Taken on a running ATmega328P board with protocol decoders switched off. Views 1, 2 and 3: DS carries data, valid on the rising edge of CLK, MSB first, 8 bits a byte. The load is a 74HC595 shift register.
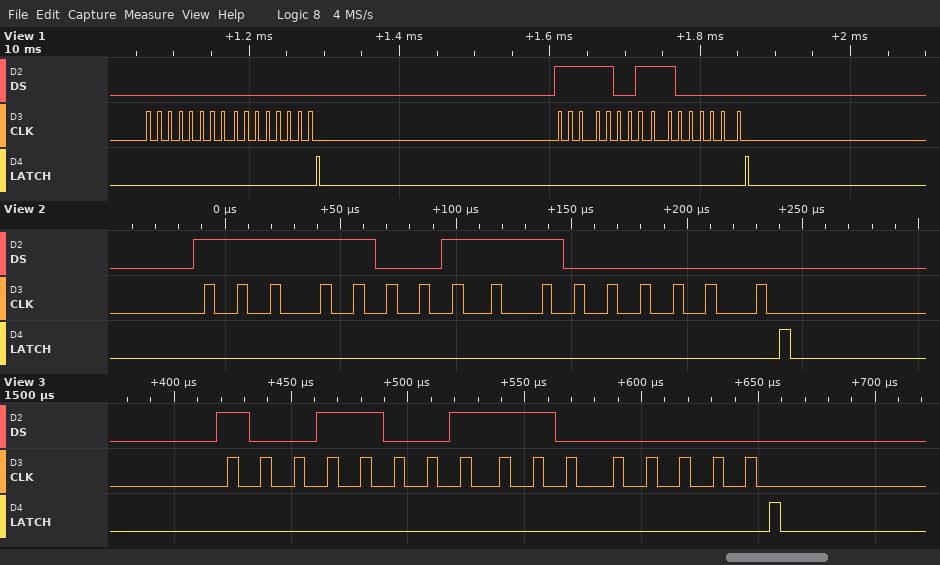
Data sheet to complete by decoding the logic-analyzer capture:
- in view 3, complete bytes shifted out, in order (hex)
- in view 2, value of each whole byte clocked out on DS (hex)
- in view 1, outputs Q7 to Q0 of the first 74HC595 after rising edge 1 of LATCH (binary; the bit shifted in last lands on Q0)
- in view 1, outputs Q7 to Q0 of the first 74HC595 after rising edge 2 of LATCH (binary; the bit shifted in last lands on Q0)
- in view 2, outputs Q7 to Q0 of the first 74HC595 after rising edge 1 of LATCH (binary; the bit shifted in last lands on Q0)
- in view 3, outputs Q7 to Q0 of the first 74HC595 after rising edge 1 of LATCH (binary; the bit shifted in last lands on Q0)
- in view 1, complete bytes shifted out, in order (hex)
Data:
99 C0
0xF9 0xC0
00000000
11000000
11000000
11000000
00 00 F9 C0
